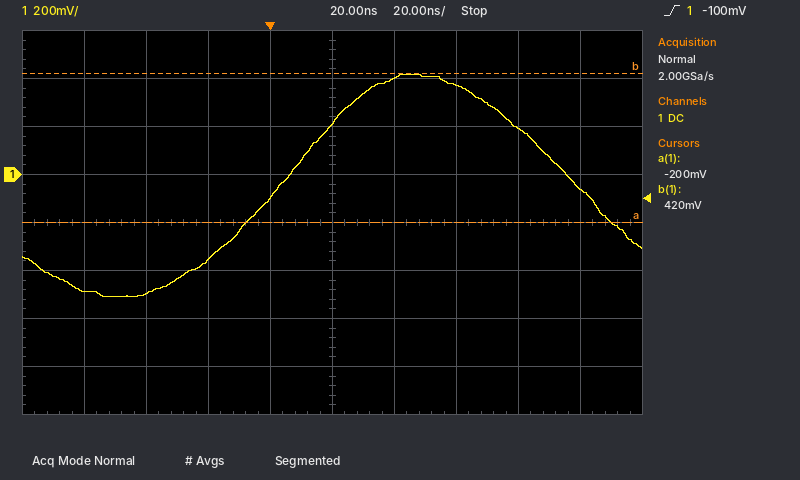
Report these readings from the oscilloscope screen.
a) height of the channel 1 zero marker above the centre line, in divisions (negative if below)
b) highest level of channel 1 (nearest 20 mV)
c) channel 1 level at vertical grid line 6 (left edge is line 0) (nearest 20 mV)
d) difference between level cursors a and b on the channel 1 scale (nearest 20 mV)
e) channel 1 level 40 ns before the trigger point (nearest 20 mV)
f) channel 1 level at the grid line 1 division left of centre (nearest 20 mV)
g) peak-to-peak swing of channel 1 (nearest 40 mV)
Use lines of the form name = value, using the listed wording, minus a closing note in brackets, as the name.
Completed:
height of the channel 1 zero marker above the centre line, in divisions = +1.0 div
highest level of channel 1 = 420 mV
channel 1 level at vertical grid line 6 (left edge is line 0) = 400 mV
difference between level cursors a and b on the channel 1 scale = 620 mV
channel 1 level 40 ns before the trigger point = -500 mV
channel 1 level at the grid line 1 division left of centre = -100 mV
peak-to-peak swing of channel 1 = 920 mV
